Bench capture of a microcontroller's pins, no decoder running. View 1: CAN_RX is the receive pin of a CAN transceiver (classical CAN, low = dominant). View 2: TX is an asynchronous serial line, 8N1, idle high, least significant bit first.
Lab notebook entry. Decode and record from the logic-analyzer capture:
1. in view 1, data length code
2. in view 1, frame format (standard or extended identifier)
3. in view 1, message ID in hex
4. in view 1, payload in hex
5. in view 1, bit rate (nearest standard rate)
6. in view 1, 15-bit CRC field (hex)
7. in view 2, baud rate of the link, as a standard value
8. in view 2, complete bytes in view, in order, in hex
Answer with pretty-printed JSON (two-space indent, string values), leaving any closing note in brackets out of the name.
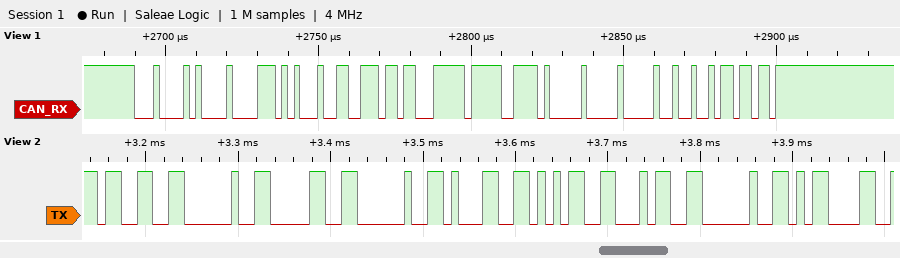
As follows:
{
  "in view 1, data length code": "8",
  "in view 1, frame format": "standard",
  "in view 1, message ID in hex": "0x10A",
  "in view 1, payload in hex": "75 13 3B 63 FF 7A 00 00",
  "in view 1, bit rate": "500 kbit/s",
  "in view 1, 15-bit CRC field": "0x496D",
  "in view 2, baud rate of the link, as a standard value": "115200 baud",
  "in view 2, complete bytes in view, in order, in hex": "33 20 30 20 31 35 34 20 0D"
}
